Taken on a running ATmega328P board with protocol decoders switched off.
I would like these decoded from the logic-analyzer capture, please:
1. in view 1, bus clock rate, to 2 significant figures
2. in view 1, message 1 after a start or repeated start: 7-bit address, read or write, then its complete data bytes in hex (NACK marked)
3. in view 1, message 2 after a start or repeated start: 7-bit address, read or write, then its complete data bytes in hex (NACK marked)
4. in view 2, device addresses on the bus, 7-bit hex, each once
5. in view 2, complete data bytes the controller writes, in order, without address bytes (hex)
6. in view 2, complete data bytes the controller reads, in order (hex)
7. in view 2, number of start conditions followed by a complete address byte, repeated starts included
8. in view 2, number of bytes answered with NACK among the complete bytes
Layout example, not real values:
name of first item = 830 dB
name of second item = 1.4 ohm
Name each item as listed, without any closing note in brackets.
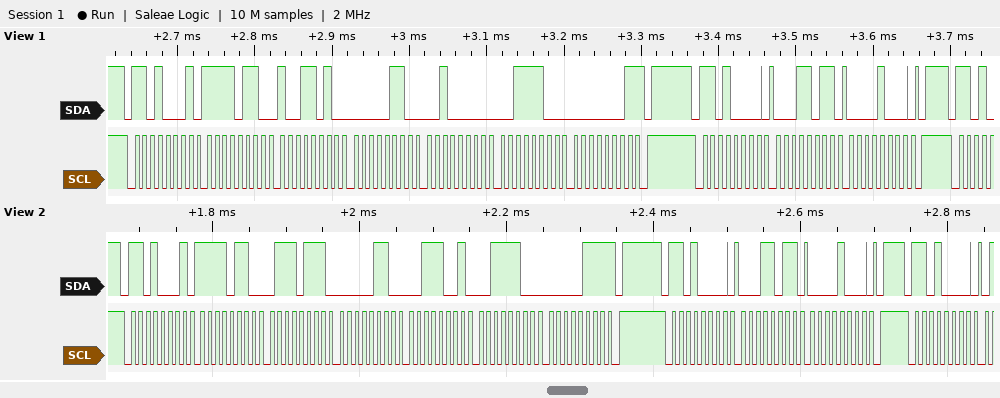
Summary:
in view 1, bus clock rate, to 2 significant figures = 100 kHz
in view 1, message 1 after a start or repeated start: 7-bit address, read or write, then its complete data bytes in hex = 0x68 read: F6 9A 06 20 3C 01 NACK
in view 1, message 2 after a start or repeated start: 7-bit address, read or write, then its complete data bytes in hex = 0x68 write: 1B 08
in view 2, device addresses on the bus, 7-bit hex, each once = 0x68
in view 2, complete data bytes the controller writes, in order, without address bytes = 1B 08
in view 2, complete data bytes the controller reads, in order = F6 77 06 39 3C 07
in view 2, number of start conditions followed by a complete address byte, repeated starts included = 3
in view 2, number of bytes answered with NACK among the complete bytes = 1
